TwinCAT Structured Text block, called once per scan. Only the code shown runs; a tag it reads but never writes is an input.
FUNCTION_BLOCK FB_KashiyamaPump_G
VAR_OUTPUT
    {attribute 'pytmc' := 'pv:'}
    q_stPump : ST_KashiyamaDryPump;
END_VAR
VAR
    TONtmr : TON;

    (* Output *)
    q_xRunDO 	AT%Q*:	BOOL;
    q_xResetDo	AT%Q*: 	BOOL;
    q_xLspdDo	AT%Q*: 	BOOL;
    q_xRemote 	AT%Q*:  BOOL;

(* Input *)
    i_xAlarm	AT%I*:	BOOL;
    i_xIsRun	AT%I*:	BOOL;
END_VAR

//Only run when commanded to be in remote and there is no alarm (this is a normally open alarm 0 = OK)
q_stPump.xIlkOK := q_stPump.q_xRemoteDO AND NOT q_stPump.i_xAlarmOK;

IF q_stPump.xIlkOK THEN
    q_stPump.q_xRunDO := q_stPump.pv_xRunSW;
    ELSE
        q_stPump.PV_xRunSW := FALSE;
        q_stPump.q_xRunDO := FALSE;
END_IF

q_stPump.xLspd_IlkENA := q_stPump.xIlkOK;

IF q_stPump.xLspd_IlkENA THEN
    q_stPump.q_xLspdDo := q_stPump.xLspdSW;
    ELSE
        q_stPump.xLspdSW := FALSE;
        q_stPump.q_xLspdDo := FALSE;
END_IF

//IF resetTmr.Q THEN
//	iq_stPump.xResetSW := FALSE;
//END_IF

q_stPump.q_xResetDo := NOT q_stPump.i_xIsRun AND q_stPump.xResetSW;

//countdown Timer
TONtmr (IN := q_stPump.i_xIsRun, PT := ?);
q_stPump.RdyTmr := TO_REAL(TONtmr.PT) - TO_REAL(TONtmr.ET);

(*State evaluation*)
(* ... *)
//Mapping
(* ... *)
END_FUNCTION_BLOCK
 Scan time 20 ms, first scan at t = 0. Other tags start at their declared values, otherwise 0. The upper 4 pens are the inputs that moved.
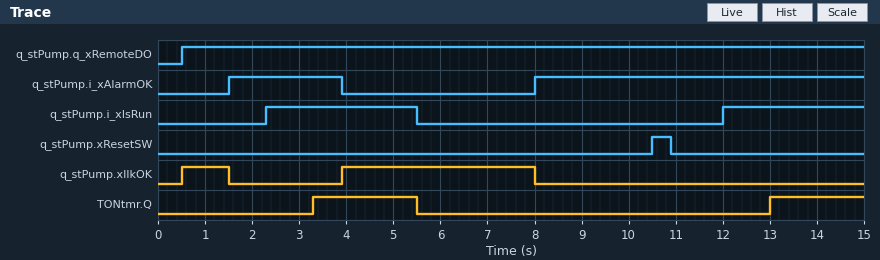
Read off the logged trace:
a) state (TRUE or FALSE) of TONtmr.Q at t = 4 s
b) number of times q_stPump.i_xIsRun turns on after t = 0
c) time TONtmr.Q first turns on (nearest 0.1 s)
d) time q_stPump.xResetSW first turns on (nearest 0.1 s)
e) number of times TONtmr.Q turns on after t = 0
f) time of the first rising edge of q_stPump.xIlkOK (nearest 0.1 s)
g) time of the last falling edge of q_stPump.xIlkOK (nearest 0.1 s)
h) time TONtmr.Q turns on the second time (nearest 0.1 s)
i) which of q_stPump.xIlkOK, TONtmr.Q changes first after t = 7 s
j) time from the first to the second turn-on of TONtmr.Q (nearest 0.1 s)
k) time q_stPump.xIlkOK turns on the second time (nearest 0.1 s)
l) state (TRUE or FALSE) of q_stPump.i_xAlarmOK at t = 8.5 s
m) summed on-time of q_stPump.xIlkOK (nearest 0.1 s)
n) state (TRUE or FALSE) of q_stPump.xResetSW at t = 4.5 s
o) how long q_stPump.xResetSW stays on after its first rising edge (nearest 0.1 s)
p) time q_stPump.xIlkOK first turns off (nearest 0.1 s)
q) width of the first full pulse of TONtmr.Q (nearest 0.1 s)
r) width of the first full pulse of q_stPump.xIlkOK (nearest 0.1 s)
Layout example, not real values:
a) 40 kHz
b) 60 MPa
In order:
a) TRUE
b) 2
c) 3.3 s
d) 10.5 s
e) 2
f) 0.5 s
g) 8.0 s
h) 13.0 s
i) q_stPump.xIlkOK
j) 9.7 s
k) 3.9 s
l) TRUE
m) 5.1 s
n) FALSE
o) 0.4 s
p) 1.5 s
q) 2.2 s
r) 1.0 s
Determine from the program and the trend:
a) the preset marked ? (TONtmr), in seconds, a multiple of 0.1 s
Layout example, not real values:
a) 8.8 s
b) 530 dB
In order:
a) 1.0 s
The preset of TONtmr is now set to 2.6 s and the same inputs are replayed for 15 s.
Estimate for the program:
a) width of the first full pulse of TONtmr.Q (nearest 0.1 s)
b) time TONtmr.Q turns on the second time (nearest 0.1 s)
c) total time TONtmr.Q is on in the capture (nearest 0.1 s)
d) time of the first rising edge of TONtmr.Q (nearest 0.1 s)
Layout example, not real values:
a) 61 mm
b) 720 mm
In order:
a) 0.6 s
b) 14.6 s
c) 1.0 s
d) 4.9 s
